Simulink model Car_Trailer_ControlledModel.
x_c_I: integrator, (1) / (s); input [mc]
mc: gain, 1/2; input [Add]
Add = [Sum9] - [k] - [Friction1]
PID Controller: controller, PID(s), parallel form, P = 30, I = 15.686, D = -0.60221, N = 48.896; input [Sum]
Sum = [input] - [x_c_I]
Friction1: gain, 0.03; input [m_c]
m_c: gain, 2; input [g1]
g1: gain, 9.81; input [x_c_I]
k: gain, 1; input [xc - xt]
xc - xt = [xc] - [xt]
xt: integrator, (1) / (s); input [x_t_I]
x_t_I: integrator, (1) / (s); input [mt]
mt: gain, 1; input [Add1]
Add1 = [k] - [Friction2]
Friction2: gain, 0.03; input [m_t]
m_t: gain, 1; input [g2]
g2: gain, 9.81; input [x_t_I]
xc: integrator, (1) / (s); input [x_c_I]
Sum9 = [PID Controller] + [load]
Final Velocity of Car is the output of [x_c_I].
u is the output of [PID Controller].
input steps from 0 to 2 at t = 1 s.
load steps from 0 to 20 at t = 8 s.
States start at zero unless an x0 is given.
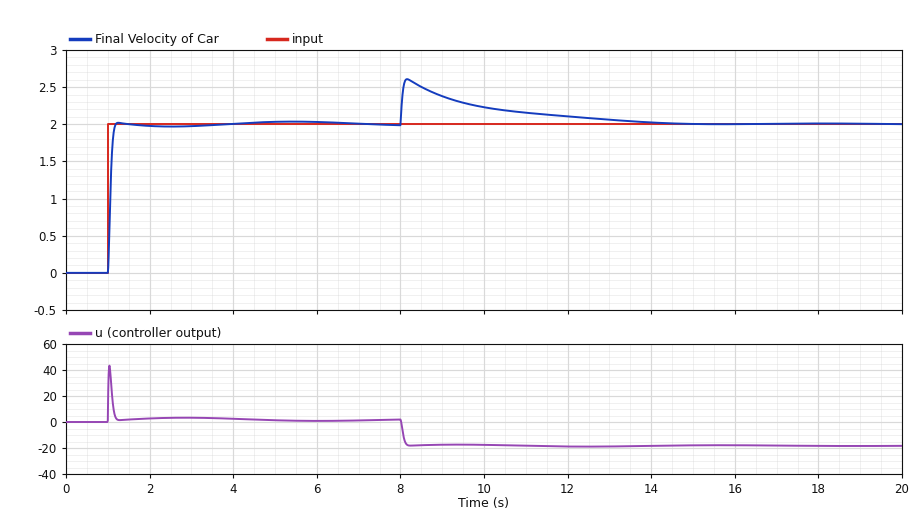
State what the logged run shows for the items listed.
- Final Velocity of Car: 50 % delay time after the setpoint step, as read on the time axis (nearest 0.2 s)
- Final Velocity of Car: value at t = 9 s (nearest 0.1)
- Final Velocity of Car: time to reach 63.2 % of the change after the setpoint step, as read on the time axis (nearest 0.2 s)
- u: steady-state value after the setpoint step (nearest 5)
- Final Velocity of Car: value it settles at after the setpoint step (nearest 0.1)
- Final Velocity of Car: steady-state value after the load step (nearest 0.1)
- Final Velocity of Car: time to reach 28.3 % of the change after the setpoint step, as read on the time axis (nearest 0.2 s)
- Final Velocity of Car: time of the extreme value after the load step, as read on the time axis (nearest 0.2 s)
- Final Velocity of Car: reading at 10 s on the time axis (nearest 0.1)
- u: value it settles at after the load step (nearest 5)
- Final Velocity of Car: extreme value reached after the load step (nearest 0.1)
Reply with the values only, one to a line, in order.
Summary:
1.0 s
2.4
1.0 s
0
2.0
2.0
1.0 s
8.2 s
2.2
-20
2.6
